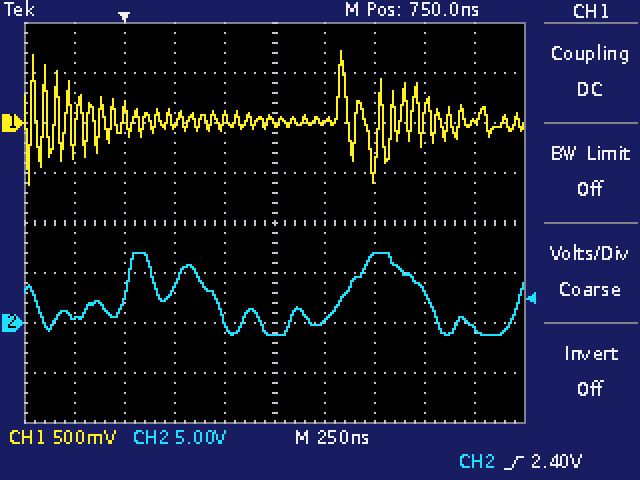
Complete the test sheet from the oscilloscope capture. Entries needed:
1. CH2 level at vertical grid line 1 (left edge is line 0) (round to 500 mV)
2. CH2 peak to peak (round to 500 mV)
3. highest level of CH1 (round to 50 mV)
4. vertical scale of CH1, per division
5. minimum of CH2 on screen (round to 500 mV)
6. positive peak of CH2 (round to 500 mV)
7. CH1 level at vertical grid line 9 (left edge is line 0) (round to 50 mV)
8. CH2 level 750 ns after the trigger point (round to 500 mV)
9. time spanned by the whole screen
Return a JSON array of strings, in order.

["500 mV", "8.0 V", "700 mV", "500 mV", "-1.0 V", "7.0 V", "0 mV", "-1.0 V", "2.5 µs"]
